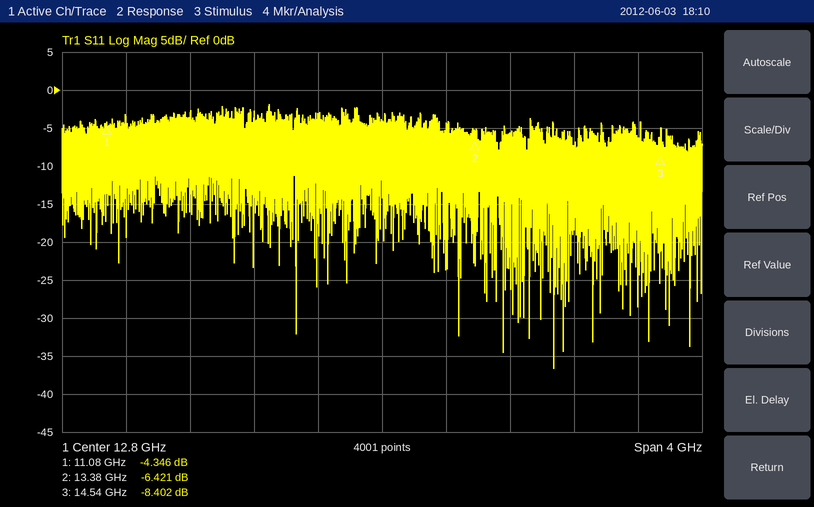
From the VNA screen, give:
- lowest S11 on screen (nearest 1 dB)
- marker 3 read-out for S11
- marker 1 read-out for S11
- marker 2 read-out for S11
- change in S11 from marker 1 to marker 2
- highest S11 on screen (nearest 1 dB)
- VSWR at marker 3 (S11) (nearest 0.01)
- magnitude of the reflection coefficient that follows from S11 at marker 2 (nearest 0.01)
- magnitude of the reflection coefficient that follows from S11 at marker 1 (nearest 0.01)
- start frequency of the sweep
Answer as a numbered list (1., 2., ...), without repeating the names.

1. -37 dB
2. -8.402 dB
3. -4.346 dB
4. -6.421 dB
5. -2.075 dB
6. -2 dB
7. 2.23
8. 0.48
9. 0.61
10. 10.8 GHz
